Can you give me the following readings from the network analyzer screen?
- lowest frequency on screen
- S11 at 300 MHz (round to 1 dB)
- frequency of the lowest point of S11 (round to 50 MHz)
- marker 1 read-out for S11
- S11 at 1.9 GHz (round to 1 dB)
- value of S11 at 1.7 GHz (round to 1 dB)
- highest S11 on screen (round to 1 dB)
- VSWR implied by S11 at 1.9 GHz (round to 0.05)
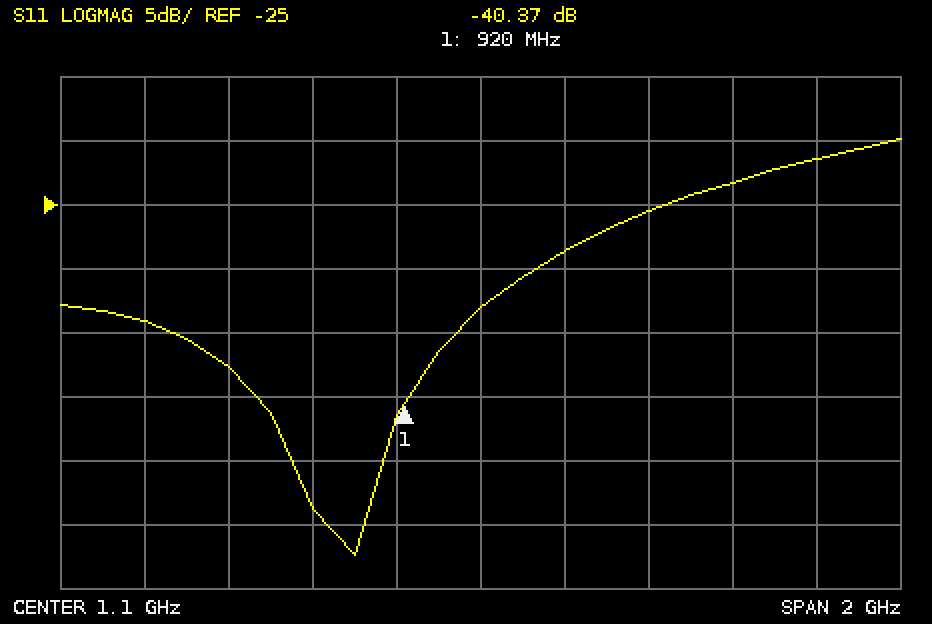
100 MHz
-34 dB
800 MHz
-40.37 dB
-21 dB
-23 dB
-20 dB
1.20
